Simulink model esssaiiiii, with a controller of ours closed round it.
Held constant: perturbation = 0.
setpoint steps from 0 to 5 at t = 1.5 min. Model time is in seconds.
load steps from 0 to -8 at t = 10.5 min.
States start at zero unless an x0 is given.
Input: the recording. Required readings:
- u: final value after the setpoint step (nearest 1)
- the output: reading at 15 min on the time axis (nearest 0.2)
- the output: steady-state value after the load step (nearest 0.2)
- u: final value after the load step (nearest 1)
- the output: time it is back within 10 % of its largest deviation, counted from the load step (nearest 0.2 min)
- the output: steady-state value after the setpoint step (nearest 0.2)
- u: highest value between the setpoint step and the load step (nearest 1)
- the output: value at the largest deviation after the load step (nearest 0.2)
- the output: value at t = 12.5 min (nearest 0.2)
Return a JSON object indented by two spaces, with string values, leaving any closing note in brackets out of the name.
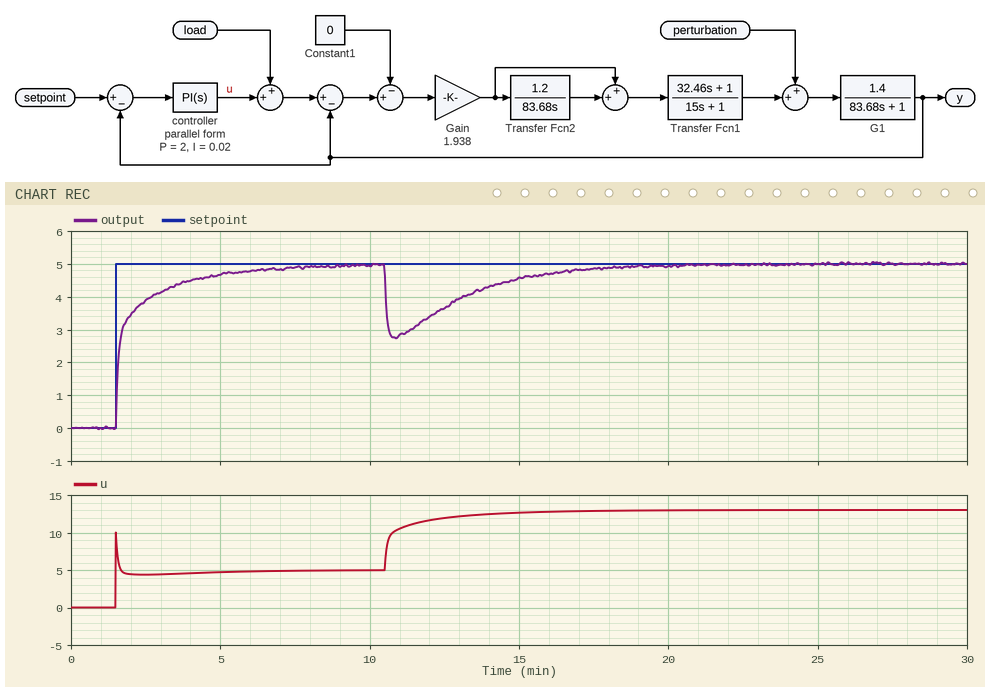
{
  "u: final value after the setpoint step": "5",
  "the output: reading at 15 min on the time axis": "4.6",
  "the output: steady-state value after the load step": "5.0",
  "u: final value after the load step": "13",
  "the output: time it is back within 10 % of its largest deviation, counted from the load step": "6.2 min",
  "the output: steady-state value after the setpoint step": "5.0",
  "u: highest value between the setpoint step and the load step": "10",
  "the output: value at the largest deviation after the load step": "2.8",
  "the output: value at t = 12.5 min": "3.6"
}
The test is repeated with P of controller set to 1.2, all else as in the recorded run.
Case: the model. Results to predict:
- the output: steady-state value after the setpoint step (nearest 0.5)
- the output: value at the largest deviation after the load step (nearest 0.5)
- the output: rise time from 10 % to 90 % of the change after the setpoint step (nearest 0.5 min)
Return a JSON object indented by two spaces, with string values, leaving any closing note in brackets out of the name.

{
  "the output: steady-state value after the setpoint step": "5.0",
  "the output: value at the largest deviation after the load step": "2.0",
  "the output: rise time from 10 % to 90 % of the change after the setpoint step": "2.5 min"
}
